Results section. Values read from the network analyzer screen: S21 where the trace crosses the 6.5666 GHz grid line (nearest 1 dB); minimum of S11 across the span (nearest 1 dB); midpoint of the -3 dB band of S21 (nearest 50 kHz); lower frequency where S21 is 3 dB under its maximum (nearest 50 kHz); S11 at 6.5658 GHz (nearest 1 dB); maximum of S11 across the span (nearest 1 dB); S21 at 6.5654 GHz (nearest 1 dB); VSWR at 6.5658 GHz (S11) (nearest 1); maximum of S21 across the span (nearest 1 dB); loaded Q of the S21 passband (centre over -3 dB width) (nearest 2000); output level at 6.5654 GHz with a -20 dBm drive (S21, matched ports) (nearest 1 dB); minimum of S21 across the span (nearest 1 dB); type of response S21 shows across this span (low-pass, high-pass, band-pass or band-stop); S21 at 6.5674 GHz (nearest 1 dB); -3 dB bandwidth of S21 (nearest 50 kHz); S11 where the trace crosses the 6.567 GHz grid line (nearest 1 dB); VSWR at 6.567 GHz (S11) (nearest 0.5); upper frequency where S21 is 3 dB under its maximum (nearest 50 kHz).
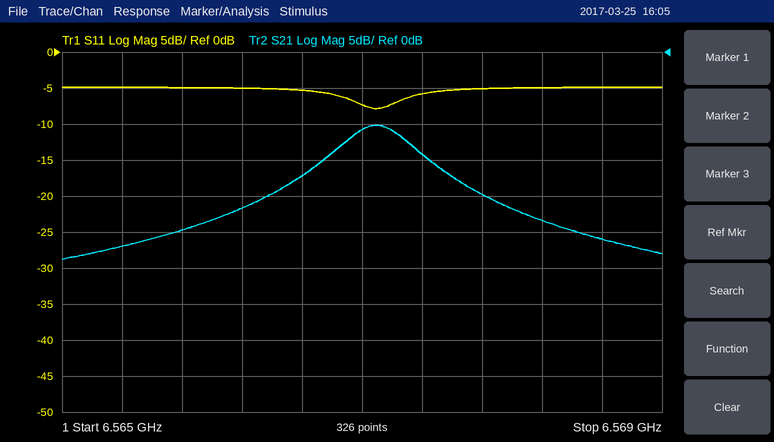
-17 dB
-8 dB
6.56710 GHz
6.56685 GHz
-5 dB
-5 dB
-27 dB
4
-10 dB
14000
-47 dBm
-29 dB
band-pass
-14 dB
500 kHz
-7 dB
2.5
6.56735 GHz
